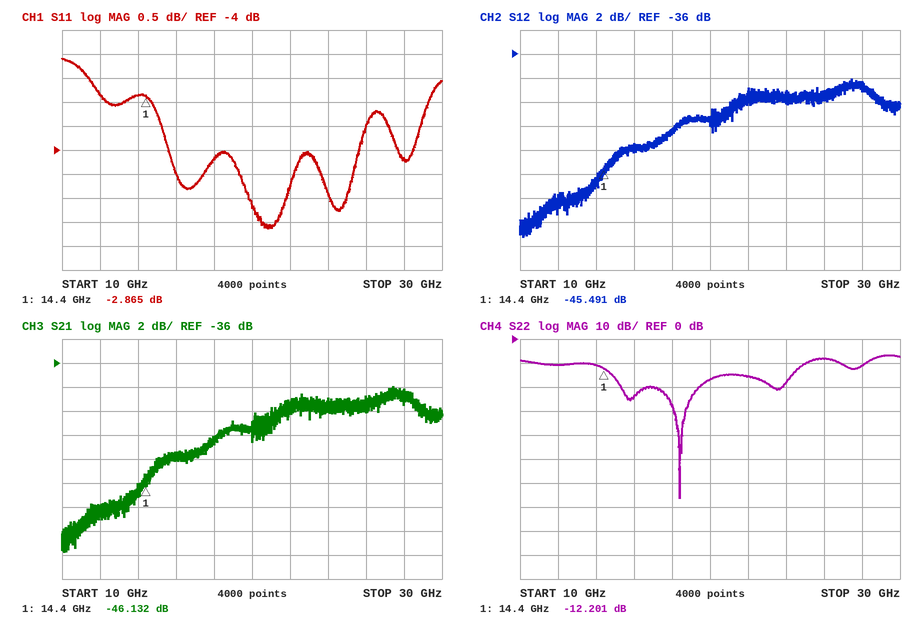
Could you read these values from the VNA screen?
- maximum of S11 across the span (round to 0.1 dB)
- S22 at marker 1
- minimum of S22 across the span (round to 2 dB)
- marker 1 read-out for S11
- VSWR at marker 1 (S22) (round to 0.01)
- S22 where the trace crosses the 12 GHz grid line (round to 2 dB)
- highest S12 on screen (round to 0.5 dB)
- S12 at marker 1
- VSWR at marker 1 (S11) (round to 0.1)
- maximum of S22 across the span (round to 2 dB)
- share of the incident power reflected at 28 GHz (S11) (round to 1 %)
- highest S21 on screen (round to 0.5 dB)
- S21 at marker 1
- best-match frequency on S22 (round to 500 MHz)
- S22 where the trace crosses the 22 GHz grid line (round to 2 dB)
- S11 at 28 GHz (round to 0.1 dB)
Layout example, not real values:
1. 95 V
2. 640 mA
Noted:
1. -2.1 dB
2. -12.201 dB
3. -66 dB
4. -2.865 dB
5. 1.65
6. -10 dB
7. -38.0 dB
8. -45.491 dB
9. 6.1
10. -6 dB
11. 38 %
12. -38.0 dB
13. -46.132 dB
14. 18.5 GHz
15. -16 dB
16. -4.2 dB
